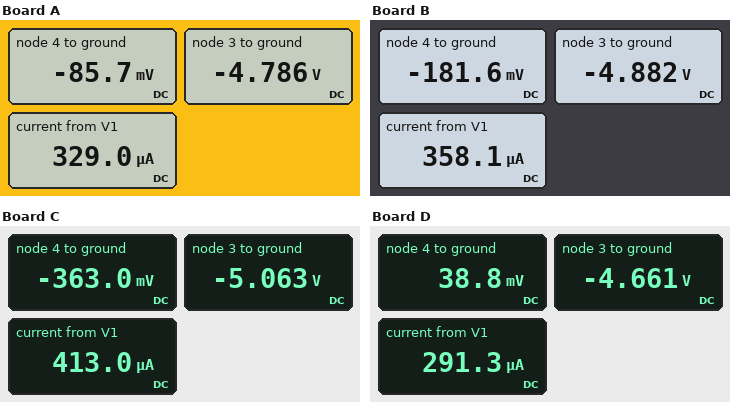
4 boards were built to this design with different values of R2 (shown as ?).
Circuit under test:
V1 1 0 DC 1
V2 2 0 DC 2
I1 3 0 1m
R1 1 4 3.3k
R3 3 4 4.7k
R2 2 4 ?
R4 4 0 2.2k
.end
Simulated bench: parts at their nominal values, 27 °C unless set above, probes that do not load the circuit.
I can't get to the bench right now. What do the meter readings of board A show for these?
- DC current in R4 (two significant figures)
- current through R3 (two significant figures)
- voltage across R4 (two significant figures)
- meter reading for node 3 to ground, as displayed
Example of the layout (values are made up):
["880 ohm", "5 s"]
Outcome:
["39 µA", "1.0 mA", "86 mV", "-4.786 V"]
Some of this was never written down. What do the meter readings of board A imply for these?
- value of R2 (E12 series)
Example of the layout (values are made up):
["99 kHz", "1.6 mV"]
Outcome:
["3.3 kΩ"]
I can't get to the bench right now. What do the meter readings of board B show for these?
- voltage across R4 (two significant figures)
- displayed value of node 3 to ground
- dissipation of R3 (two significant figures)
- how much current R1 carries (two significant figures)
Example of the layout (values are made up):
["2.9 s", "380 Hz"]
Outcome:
["180 mV", "-4.882 V", "4.7 mW", "360 µA"]
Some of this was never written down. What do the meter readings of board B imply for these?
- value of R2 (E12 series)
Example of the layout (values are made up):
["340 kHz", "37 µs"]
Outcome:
["3.9 kΩ"]
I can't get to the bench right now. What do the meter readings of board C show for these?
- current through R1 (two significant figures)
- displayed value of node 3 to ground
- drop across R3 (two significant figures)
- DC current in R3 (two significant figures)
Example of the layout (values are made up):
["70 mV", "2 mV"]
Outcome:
["410 µA", "-5.063 V", "4.7 V", "1.0 mA"]
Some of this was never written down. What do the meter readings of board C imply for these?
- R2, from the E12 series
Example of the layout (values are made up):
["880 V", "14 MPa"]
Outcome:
["5.6 kΩ"]
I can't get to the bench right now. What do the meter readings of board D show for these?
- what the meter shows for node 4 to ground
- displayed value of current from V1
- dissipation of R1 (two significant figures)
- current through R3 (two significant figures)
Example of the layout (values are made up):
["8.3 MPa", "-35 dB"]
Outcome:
["38.8 mV", "291.3 µA", "280 µW", "1.0 mA"]
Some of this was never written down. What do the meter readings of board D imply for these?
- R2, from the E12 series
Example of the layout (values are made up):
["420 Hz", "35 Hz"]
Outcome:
["2.7 kΩ"]
